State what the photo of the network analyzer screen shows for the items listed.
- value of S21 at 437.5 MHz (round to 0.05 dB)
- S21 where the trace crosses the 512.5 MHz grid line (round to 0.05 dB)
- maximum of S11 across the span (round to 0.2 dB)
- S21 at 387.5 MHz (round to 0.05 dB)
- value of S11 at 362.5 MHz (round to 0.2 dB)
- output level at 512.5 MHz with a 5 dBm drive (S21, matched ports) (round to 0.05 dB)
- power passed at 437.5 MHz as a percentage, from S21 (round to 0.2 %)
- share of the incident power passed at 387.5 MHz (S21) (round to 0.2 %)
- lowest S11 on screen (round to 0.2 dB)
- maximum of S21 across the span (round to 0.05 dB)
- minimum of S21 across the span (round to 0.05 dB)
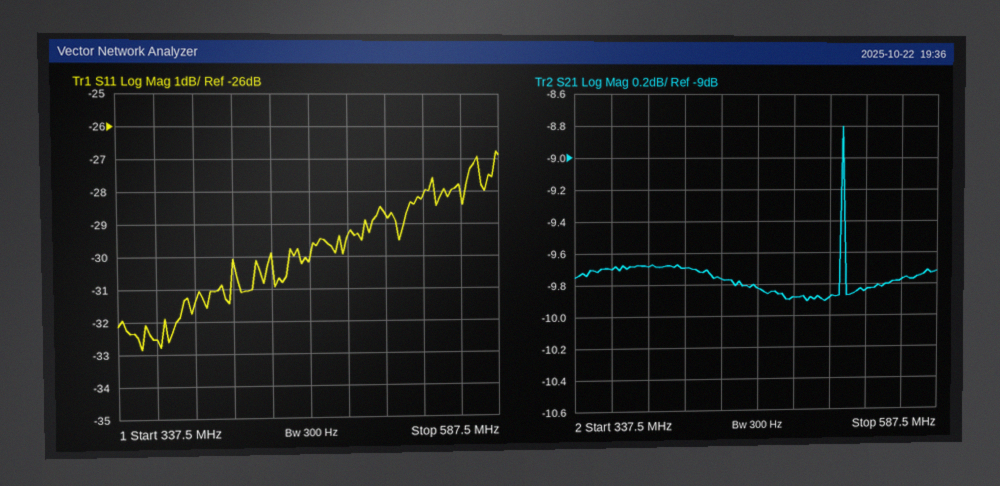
-9.75 dB
-9.90 dB
-26.8 dB
-9.70 dB
-32.6 dB
-4.90 dBm
10.6 %
10.8 %
-32.8 dB
-8.80 dB
-9.90 dB
